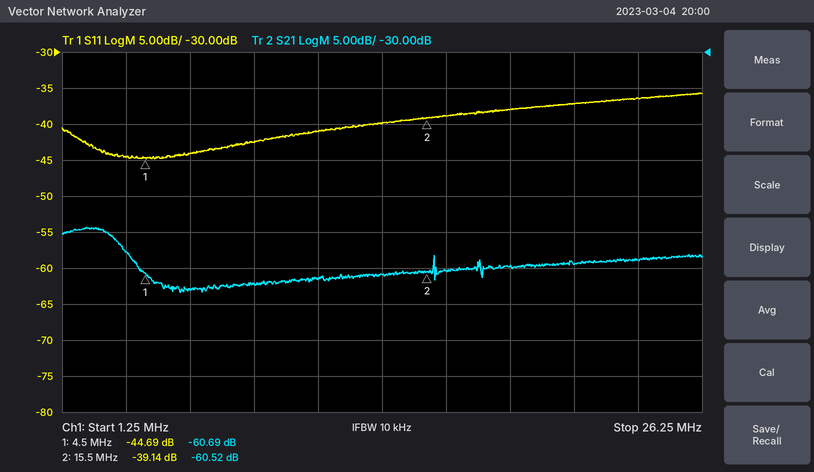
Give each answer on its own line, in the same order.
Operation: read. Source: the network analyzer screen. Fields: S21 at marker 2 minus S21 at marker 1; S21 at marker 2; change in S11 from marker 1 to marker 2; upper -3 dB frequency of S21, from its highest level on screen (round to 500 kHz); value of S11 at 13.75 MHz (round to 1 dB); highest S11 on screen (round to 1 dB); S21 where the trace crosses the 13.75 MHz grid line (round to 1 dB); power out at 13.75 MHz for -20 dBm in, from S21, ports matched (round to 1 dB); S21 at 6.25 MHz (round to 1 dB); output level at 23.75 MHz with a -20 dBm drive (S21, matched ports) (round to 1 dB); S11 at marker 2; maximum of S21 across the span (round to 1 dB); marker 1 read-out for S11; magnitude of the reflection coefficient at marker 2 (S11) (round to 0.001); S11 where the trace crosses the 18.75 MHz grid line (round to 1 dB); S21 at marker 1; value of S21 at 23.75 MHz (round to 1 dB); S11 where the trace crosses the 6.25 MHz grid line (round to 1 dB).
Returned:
0.17 dB
-60.52 dB
5.55 dB
3.5 MHz
-40 dB
-36 dB
-61 dB
-81 dBm
-63 dB
-79 dBm
-39.14 dB
-54 dB
-44.69 dB
0.011
-38 dB
-60.69 dB
-59 dB
-44 dB
